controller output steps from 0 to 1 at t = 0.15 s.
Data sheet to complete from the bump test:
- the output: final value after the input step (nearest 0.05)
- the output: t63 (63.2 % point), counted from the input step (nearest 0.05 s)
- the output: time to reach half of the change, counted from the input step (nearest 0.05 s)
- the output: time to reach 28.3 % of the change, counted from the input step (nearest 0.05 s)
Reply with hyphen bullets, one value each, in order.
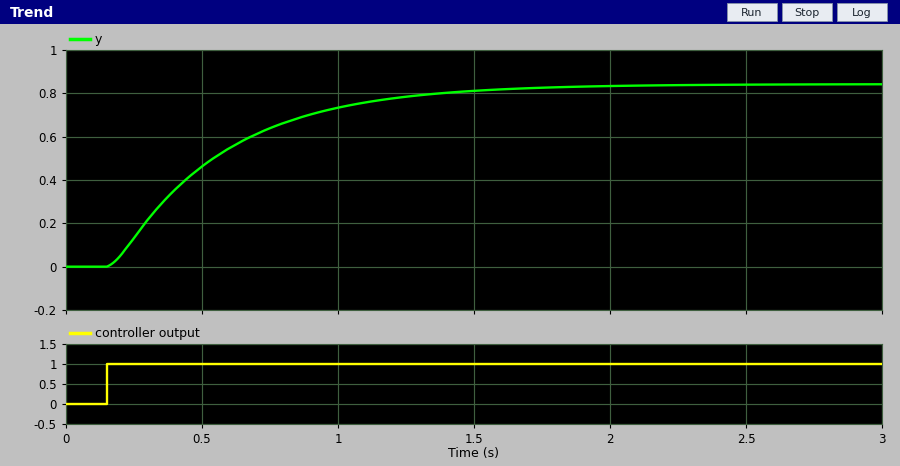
- 0.85
- 0.45 s
- 0.30 s
- 0.15 s
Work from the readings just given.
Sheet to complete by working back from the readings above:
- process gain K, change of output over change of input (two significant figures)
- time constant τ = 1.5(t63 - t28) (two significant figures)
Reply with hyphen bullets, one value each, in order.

- 0.85
- 0.45 s
